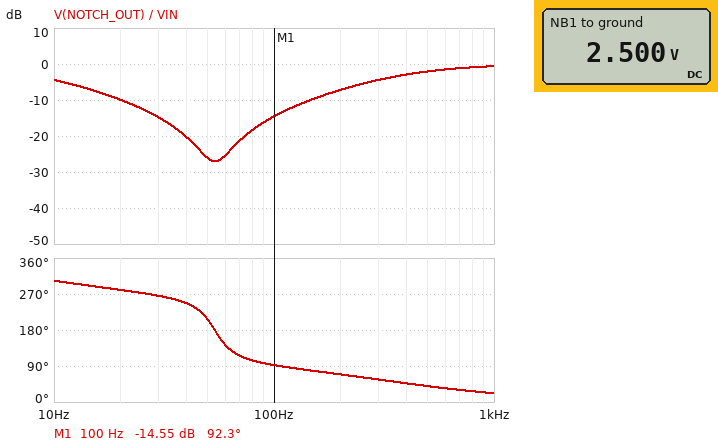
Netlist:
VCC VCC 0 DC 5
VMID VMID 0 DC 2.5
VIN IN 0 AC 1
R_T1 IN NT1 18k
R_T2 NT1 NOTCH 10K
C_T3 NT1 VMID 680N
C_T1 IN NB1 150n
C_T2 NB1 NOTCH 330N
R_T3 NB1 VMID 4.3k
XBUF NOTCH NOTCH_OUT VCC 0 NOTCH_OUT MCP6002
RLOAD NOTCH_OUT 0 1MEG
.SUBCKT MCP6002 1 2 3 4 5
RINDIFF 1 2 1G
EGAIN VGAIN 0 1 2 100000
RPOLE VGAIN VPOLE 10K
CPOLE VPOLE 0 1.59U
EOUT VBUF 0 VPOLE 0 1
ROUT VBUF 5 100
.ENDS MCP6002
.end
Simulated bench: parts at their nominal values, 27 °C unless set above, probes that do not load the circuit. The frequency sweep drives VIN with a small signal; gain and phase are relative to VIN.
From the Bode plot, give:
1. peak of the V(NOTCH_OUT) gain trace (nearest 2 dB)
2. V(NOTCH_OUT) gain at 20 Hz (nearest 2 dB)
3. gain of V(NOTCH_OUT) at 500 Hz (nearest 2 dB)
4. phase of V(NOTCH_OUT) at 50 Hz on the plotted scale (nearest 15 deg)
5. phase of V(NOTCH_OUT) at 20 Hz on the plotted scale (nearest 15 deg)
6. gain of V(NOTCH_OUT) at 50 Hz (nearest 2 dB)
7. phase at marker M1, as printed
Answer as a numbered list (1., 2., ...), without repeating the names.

1. 0 dB
2. -10 dB
3. -2 dB
4. 210 deg
5. 285 deg
6. -26 dB
7. 92.3 deg
